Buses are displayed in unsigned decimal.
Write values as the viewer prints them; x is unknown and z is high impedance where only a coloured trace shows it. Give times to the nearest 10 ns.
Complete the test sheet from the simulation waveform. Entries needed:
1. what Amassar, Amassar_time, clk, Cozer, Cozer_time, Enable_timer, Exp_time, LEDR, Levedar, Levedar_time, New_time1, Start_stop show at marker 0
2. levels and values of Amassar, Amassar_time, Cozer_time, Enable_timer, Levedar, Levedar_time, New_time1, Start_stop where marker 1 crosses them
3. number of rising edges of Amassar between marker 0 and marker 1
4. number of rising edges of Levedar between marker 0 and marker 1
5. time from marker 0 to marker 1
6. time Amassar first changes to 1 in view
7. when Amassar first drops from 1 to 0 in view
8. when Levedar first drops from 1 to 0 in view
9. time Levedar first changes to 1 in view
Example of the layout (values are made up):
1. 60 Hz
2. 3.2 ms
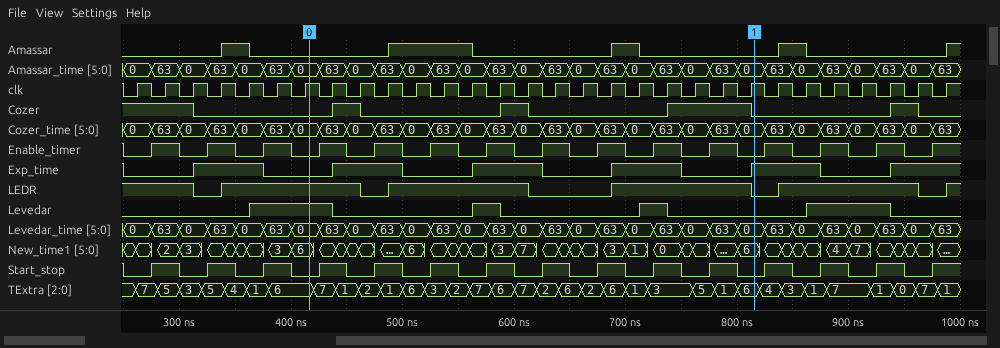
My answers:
1. Amassar=0, Amassar_time=0, clk=1, Cozer=0, Cozer_time=0, Enable_timer=0, Exp_time=0, LEDR=1, Levedar=1, Levedar_time=0, New_time1=6, Start_stop=0
2. Amassar=0, Amassar_time=0, Cozer_time=0, Enable_timer=0, Levedar=0, Levedar_time=0, New_time1=6, Start_stop=0
3. 2
4. 2
5. 400 ns
6. 340 ns
7. 360 ns
8. 440 ns
9. 360 ns
